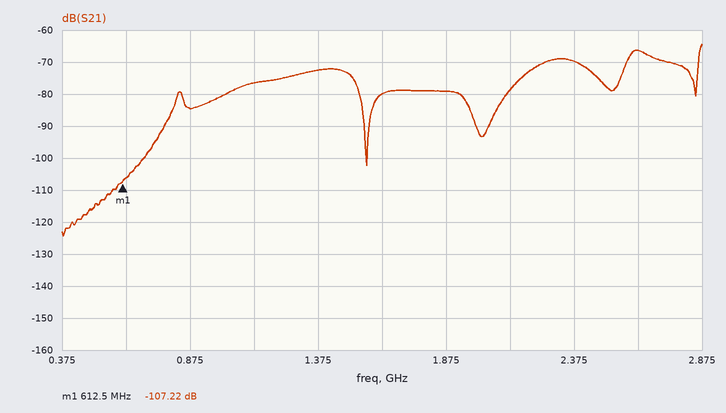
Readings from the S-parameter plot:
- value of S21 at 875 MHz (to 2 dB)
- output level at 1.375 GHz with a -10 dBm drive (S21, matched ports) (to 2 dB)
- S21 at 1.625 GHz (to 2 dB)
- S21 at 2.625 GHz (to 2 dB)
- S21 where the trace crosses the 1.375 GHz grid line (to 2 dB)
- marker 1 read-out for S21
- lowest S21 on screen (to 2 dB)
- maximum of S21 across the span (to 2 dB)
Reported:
-84 dB
-82 dBm
-80 dB
-66 dB
-72 dB
-107.22 dB
-124 dB
-64 dB
